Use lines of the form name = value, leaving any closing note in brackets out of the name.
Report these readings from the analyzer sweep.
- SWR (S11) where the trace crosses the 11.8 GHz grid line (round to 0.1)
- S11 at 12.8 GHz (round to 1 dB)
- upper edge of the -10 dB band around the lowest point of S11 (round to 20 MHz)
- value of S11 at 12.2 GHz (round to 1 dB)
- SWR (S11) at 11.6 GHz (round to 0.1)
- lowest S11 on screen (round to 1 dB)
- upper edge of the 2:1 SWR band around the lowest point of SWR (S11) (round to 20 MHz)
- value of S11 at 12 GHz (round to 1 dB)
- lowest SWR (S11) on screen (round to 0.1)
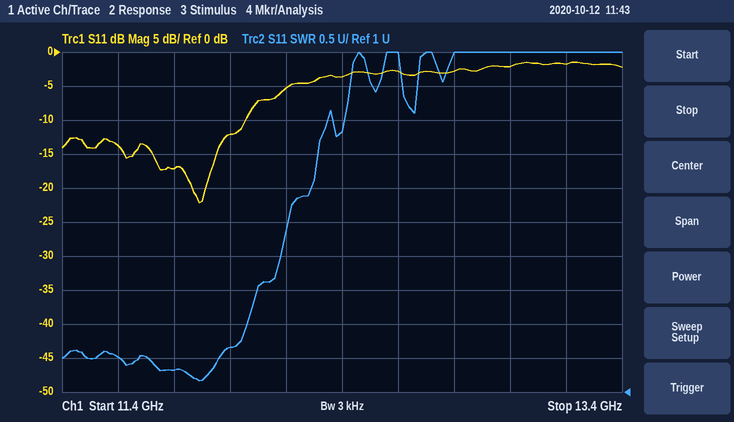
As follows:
SWR (S11) where the trace crosses the 11.8 GHz grid line = 1.3
S11 at 12.8 GHz = -3 dB
upper edge of the -10 dB band around the lowest point of S11 = 12.06 GHz
value of S11 at 12.2 GHz = -5 dB
SWR (S11) at 11.6 GHz = 1.5
lowest S11 on screen = -22 dB
upper edge of the 2:1 SWR band around the lowest point of SWR (S11) = 12.06 GHz
value of S11 at 12 GHz = -12 dB
lowest SWR (S11) on screen = 1.2
